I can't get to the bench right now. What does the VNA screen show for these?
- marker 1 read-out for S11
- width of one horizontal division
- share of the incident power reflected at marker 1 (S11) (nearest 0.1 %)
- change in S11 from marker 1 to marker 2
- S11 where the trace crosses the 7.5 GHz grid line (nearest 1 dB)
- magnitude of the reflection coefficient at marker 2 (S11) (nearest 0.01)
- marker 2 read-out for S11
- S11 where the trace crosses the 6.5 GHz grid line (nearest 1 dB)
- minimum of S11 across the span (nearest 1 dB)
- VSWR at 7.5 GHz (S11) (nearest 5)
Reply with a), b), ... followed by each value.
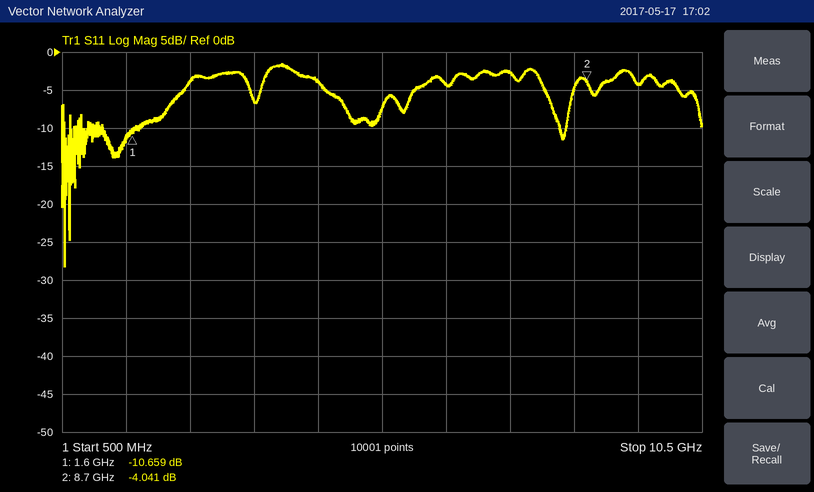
a) -10.659 dB
b) 1 GHz
c) 8.6 %
d) 6.618 dB
e) -3 dB
f) 0.63
g) -4.041 dB
h) -4 dB
i) -28 dB
j) 5
